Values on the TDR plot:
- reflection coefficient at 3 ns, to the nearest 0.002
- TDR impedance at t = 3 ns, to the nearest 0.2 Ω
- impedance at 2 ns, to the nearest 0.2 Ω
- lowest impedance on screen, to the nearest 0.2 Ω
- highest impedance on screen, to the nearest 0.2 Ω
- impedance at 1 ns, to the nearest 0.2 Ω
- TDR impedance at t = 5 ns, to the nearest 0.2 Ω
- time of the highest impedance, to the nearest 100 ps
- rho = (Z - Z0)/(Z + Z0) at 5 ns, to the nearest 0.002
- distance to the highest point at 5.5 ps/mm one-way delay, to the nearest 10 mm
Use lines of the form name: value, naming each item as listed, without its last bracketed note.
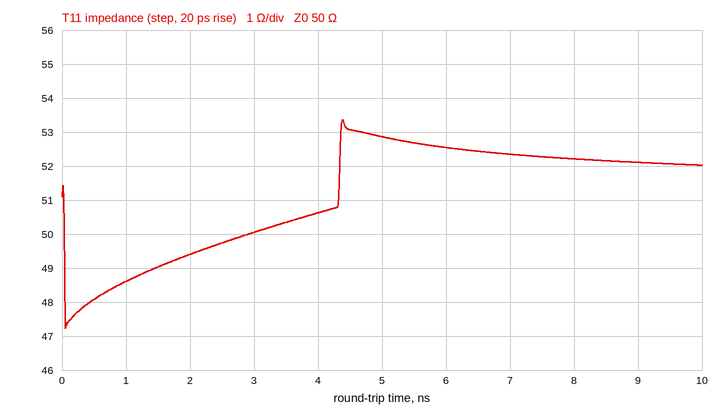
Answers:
reflection coefficient at 3 ns, to the nearest 0.002: 0.000
TDR impedance at t = 3 ns, to the nearest 0.2 Ω: 50.0 Ω
impedance at 2 ns, to the nearest 0.2 Ω: 49.4 Ω
lowest impedance on screen, to the nearest 0.2 Ω: 47.2 Ω
highest impedance on screen, to the nearest 0.2 Ω: 53.4 Ω
impedance at 1 ns, to the nearest 0.2 Ω: 48.6 Ω
TDR impedance at t = 5 ns, to the nearest 0.2 Ω: 52.8 Ω
time of the highest impedance, to the nearest 100 ps: 4.4 ns
rho = (Z - Z0)/(Z + Z0) at 5 ns, to the nearest 0.002: +0.028
distance to the highest point at 5.5 ps/mm one-way delay, to the nearest 10 mm: 400 mm
